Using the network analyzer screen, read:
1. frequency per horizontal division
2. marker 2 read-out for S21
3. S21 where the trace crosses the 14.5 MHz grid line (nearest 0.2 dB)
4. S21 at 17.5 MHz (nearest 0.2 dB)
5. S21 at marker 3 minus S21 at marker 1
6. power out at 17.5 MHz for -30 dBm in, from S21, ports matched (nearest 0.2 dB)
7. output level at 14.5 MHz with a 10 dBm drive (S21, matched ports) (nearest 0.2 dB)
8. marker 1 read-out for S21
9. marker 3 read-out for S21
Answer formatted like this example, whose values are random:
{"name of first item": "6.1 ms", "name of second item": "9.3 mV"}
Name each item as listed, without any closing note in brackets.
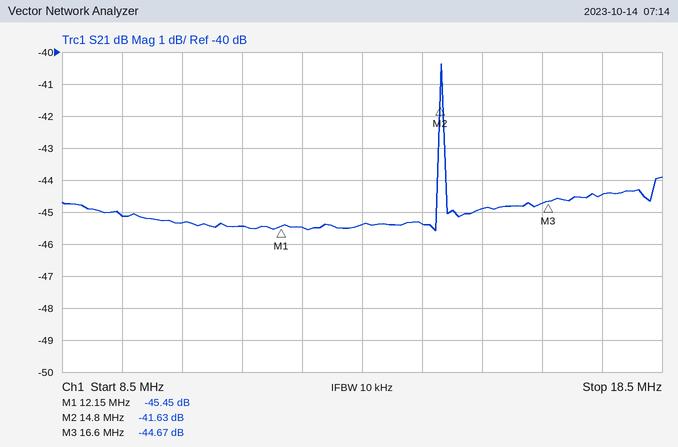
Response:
{"frequency per horizontal division": "1 MHz", "marker 2 read-out for S21": "-41.63 dB", "S21 where the trace crosses the 14.5 MHz grid line": "-45.4 dB", "S21 at 17.5 MHz": "-44.4 dB", "S21 at marker 3 minus S21 at marker 1": "0.78 dB", "power out at 17.5 MHz for -30 dBm in, from S21, ports matched": "-74.4 dBm", "output level at 14.5 MHz with a 10 dBm drive (S21, matched ports)": "-35.4 dBm", "marker 1 read-out for S21": "-45.45 dB", "marker 3 read-out for S21": "-44.67 dB"}
